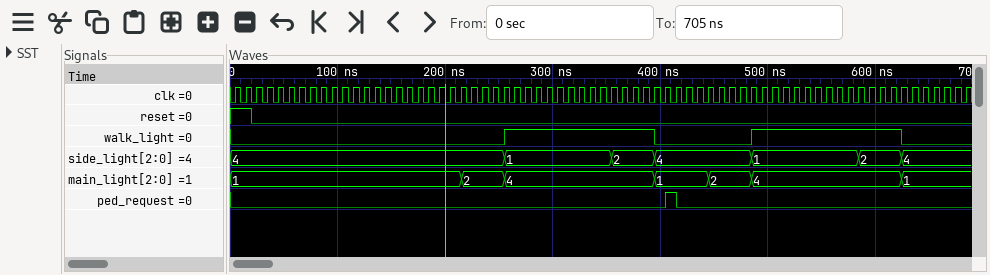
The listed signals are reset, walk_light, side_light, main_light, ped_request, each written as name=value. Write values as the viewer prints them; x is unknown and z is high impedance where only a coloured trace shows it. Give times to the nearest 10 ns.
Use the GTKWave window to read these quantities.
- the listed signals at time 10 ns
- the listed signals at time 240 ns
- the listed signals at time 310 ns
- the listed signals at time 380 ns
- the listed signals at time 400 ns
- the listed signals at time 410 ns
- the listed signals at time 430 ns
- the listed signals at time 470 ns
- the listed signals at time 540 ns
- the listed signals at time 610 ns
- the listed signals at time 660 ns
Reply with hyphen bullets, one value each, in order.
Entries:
- reset=1, walk_light=0, side_light=4, main_light=1, ped_request=0
- reset=0, walk_light=0, side_light=4, main_light=2, ped_request=0
- reset=0, walk_light=1, side_light=1, main_light=4, ped_request=0
- reset=0, walk_light=1, side_light=2, main_light=4, ped_request=0
- reset=0, walk_light=0, side_light=4, main_light=1, ped_request=0
- reset=0, walk_light=0, side_light=4, main_light=1, ped_request=1
- reset=0, walk_light=0, side_light=4, main_light=1, ped_request=0
- reset=0, walk_light=0, side_light=4, main_light=2, ped_request=0
- reset=0, walk_light=1, side_light=1, main_light=4, ped_request=0
- reset=0, walk_light=1, side_light=2, main_light=4, ped_request=0
- reset=0, walk_light=0, side_light=4, main_light=1, ped_request=0
